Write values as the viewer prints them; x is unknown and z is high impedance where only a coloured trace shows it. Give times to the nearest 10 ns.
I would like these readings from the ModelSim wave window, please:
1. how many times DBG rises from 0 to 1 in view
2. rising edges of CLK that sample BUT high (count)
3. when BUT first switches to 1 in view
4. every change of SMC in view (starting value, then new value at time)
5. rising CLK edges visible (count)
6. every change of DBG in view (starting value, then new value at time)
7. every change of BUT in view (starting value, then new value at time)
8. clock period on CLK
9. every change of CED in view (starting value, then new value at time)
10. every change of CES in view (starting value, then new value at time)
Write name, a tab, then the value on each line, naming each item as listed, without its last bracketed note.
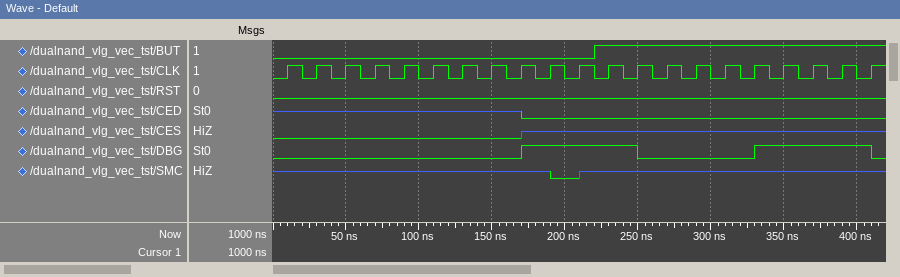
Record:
how many times DBG rises from 0 to 1 in view	2
rising edges of CLK that sample BUT high	10
when BUT first switches to 1 in view	220 ns
every change of SMC in view	z, 0 at 190 ns, z at 210 ns
rising CLK edges visible	21
every change of DBG in view	0, 1 at 170 ns, 0 at 250 ns, 1 at 330 ns, 0 at 410 ns
every change of BUT in view	0, 1 at 220 ns
clock period on CLK	20 ns
every change of CED in view	z, 0 at 170 ns
every change of CES in view	0, z at 170 ns
